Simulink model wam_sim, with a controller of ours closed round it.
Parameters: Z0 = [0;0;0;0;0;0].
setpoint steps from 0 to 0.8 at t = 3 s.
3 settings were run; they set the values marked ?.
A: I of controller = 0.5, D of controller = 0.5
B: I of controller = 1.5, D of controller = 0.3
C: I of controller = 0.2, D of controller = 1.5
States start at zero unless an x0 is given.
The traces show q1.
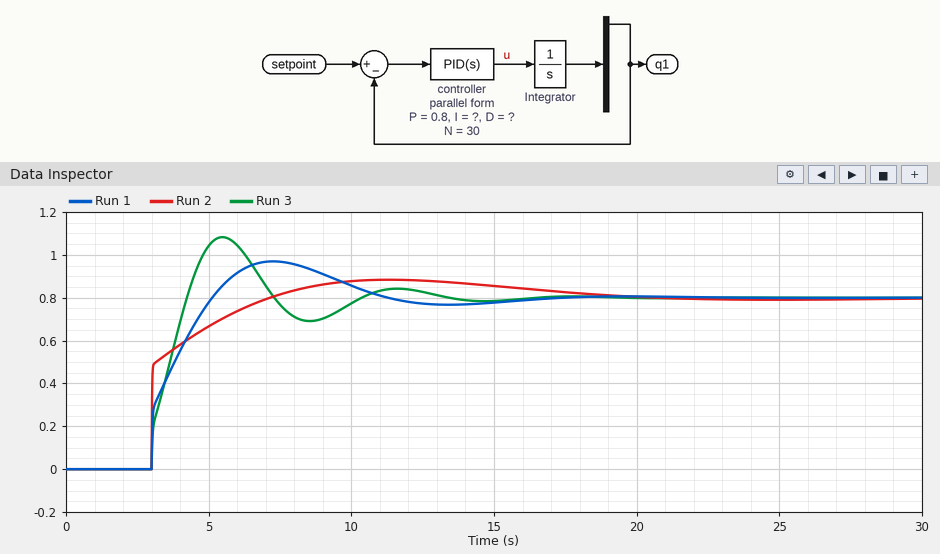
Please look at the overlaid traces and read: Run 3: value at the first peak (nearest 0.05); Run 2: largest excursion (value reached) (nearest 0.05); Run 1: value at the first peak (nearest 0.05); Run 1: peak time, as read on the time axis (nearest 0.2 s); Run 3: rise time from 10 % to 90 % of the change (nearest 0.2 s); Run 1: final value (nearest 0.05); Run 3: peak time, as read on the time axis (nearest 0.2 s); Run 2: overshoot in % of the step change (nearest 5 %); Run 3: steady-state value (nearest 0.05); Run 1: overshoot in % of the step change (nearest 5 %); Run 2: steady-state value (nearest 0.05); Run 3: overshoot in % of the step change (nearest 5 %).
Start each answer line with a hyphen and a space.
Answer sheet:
- 1.10
- 0.90
- 0.95
- 7.2 s
- 1.0 s
- 0.80
- 5.4 s
- 10 %
- 0.80
- 20 %
- 0.80
- 35 %
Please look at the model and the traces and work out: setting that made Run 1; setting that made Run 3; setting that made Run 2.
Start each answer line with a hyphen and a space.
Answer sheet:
- A
- B
- C
